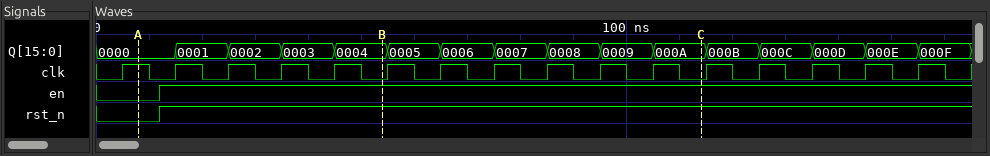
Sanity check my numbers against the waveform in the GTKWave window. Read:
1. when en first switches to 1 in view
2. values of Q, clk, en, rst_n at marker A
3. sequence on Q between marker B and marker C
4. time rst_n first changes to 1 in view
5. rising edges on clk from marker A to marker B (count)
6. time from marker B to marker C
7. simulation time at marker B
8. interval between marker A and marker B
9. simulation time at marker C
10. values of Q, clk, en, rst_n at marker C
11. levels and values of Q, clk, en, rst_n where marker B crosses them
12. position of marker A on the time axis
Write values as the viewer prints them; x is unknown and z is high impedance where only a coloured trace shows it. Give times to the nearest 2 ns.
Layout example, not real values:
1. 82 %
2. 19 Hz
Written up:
1. 12 ns
2. Q=0000, clk=1, en=0, rst_n=0
3. 0004, 0005, 0006, 0007, 0008, 0009, 000A
4. 12 ns
5. 4
6. 60 ns
7. 54 ns
8. 46 ns
9. 114 ns
10. Q=000A, clk=0, en=1, rst_n=1
11. Q=0004, clk=0, en=1, rst_n=1
12. 8 ns
